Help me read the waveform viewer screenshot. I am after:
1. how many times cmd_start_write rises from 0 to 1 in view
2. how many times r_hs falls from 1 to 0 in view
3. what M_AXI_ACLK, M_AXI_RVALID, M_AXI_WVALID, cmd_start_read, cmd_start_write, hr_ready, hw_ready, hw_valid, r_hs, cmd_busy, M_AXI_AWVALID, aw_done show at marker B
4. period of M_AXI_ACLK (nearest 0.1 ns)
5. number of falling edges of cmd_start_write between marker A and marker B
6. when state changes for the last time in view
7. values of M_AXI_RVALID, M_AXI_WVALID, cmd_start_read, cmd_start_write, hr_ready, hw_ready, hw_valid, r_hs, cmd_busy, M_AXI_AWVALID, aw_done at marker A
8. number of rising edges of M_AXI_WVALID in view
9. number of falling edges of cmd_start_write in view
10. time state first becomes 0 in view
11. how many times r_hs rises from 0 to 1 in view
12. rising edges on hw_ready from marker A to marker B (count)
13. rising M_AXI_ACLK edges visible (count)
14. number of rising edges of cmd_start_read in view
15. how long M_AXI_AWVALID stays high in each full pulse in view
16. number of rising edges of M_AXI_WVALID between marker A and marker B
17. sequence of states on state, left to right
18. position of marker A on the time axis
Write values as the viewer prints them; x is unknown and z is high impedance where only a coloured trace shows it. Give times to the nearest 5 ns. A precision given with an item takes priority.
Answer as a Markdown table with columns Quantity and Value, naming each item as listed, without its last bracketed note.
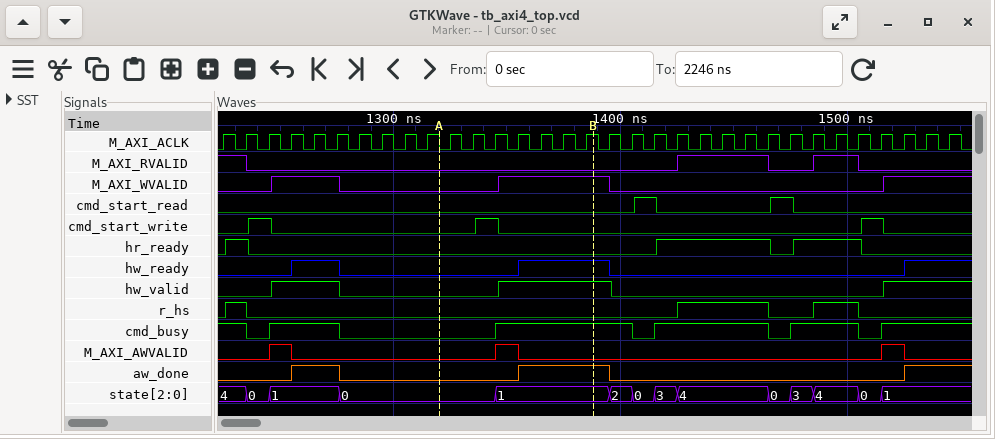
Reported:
| Quantity | Value |
|---|---|
| how many times cmd_start_write rises from 0 to 1 in view | 3 |
| how many times r_hs falls from 1 to 0 in view | 3 |
| what M_AXI_ACLK, M_AXI_RVALID, M_AXI_WVALID, cmd_start_read, cmd_start_write, hr_ready, hw_ready, hw_valid, r_hs, cmd_busy, M_AXI_AWVALID, aw_done show at marker B | M_AXI_ACLK=1, M_AXI_RVALID=0, M_AXI_WVALID=1, cmd_start_read=0, cmd_start_write=0, hr_ready=0, hw_ready=1, hw_valid=1, r_hs=0, cmd_busy=1, M_AXI_AWVALID=0, aw_done=1 |
| period of M_AXI_ACLK | 10 ns |
| number of falling edges of cmd_start_write between marker A and marker B | 1 |
| when state changes for the last time in view | 1515 ns |
| values of M_AXI_RVALID, M_AXI_WVALID, cmd_start_read, cmd_start_write, hr_ready, hw_ready, hw_valid, r_hs, cmd_busy, M_AXI_AWVALID, aw_done at marker A | M_AXI_RVALID=0, M_AXI_WVALID=0, cmd_start_read=0, cmd_start_write=0, hr_ready=0, hw_ready=0, hw_valid=0, r_hs=0, cmd_busy=0, M_AXI_AWVALID=0, aw_done=0 |
| number of rising edges of M_AXI_WVALID in view | 3 |
| number of falling edges of cmd_start_write in view | 3 |
| time state first becomes 0 in view | 1235 ns |
| how many times r_hs rises from 0 to 1 in view | 3 |
| rising edges on hw_ready from marker A to marker B | 1 |
| rising M_AXI_ACLK edges visible | 33 |
| number of rising edges of cmd_start_read in view | 2 |
| how long M_AXI_AWVALID stays high in each full pulse in view | 10 ns, 10 ns, 10 ns |
| number of rising edges of M_AXI_WVALID between marker A and marker B | 1 |
| sequence of states on state, left to right | 4, 0, 1, 0, 1, 2, 0, 3, 4, 0, 3, 4, 0, 1 |
| position of marker A on the time axis | 1320 ns |
